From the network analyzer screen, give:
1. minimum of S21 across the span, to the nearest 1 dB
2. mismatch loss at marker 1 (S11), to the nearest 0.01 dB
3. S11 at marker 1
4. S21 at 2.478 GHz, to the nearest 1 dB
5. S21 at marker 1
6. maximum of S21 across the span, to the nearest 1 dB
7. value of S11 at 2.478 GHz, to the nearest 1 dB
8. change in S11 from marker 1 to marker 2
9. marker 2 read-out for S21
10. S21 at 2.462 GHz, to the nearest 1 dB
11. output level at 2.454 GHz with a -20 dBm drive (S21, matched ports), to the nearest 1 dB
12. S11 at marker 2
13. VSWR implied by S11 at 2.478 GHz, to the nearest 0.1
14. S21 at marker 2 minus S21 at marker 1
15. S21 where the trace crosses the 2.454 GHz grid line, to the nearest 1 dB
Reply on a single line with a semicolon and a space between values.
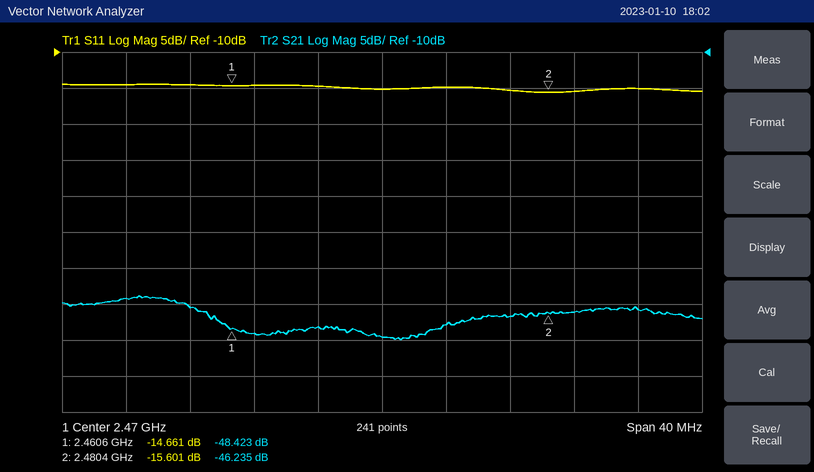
-50 dB; 0.15 dB; -14.661 dB; -47 dB; -48.423 dB; -44 dB; -15 dB; -0.940 dB; -46.235 dB; -49 dB; -64 dBm; -15.601 dB; 1.4; 2.188 dB; -44 dB
